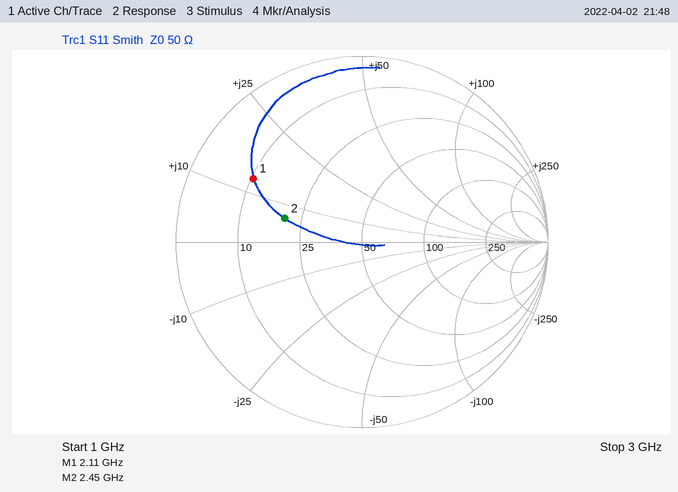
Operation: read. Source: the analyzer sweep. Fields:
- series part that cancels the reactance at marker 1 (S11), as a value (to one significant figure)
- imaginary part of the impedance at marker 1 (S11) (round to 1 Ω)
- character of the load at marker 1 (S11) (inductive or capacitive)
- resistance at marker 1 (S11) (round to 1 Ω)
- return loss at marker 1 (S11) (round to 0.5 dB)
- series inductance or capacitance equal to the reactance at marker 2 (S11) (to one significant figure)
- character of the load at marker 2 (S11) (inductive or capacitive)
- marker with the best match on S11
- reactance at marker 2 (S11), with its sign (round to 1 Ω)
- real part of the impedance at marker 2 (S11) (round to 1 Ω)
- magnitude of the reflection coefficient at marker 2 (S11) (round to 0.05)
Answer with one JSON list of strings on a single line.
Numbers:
["6 pF", "+13 Ω", "inductive", "10 Ω", "3.5 dB", "400 pH", "inductive", "marker 2", "+6 Ω", "20 Ω", "0.45"]
